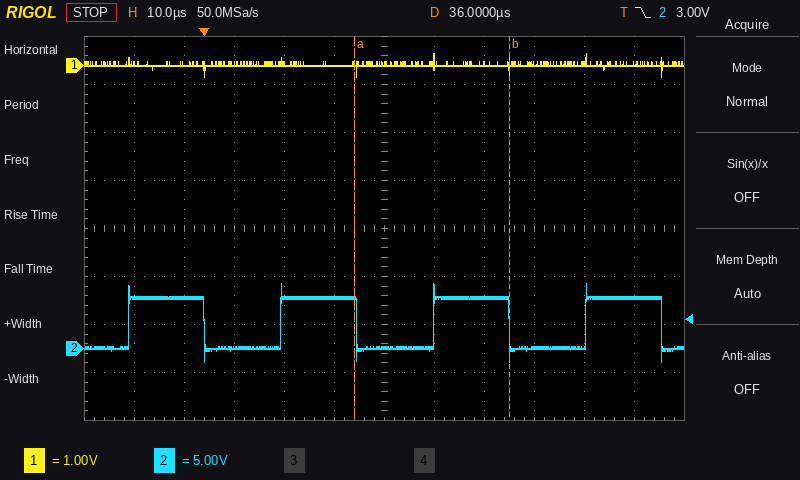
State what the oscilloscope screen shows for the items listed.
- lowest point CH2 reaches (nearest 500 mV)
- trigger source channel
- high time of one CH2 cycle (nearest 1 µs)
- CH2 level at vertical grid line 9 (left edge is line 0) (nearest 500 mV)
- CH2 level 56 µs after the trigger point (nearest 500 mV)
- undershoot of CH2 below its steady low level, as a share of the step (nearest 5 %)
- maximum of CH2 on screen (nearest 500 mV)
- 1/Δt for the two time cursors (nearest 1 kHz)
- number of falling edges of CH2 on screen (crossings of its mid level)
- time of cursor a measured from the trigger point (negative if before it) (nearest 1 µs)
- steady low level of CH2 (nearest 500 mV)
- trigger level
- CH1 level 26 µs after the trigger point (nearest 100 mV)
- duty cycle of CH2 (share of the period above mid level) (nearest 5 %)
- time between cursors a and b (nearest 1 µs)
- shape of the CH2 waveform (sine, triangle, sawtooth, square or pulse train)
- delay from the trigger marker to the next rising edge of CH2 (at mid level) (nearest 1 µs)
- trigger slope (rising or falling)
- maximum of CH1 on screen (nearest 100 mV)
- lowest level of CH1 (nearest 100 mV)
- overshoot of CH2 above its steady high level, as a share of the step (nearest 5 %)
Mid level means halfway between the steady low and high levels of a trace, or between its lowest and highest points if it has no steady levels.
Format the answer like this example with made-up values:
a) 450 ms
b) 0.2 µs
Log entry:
a) -1.5 V
b) CH2
c) 15 µs
d) 0.0 V
e) 5.5 V
f) 30 %
g) 7.0 V
h) 32 kHz
i) 4
j) +30 µs
k) 0.0 V
l) 3.00 V
m) 0.0 V
n) 50 %
o) 31 µs
p) square
q) 15 µs
r) falling
s) 200 mV
t) -200 mV
u) 30 %
